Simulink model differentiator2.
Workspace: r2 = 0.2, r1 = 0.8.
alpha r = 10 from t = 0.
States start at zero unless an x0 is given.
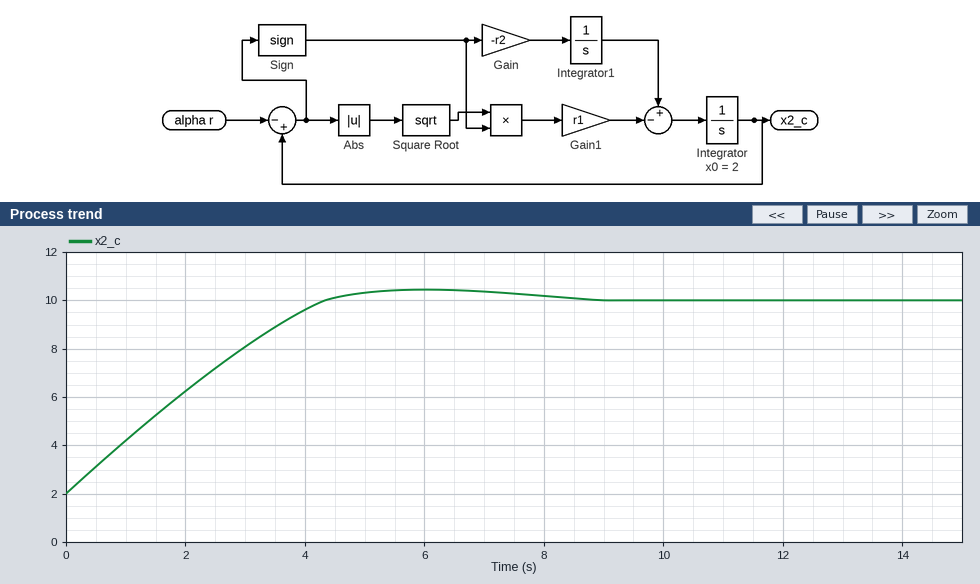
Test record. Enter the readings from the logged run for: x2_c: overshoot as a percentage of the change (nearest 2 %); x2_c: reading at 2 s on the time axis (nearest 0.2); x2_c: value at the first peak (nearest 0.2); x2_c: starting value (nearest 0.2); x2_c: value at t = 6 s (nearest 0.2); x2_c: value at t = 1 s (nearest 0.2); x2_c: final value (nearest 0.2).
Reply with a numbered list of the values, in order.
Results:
1. 6 %
2. 6.2
3. 10.4
4. 2.0
5. 10.4
6. 4.2
7. 10.0
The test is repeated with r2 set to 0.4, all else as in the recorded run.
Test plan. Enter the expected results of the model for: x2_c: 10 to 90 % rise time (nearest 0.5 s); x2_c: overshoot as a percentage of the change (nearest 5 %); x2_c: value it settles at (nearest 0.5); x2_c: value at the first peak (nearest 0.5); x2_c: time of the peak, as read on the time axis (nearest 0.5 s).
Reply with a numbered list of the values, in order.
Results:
1. 3.0 s
2. 10 %
3. 10.0
4. 11.0
5. 5.5 s
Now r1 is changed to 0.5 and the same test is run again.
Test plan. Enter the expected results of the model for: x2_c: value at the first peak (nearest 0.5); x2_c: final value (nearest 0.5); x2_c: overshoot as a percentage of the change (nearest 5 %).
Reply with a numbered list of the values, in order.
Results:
1. 11.0
2. 10.0
3. 15 %
